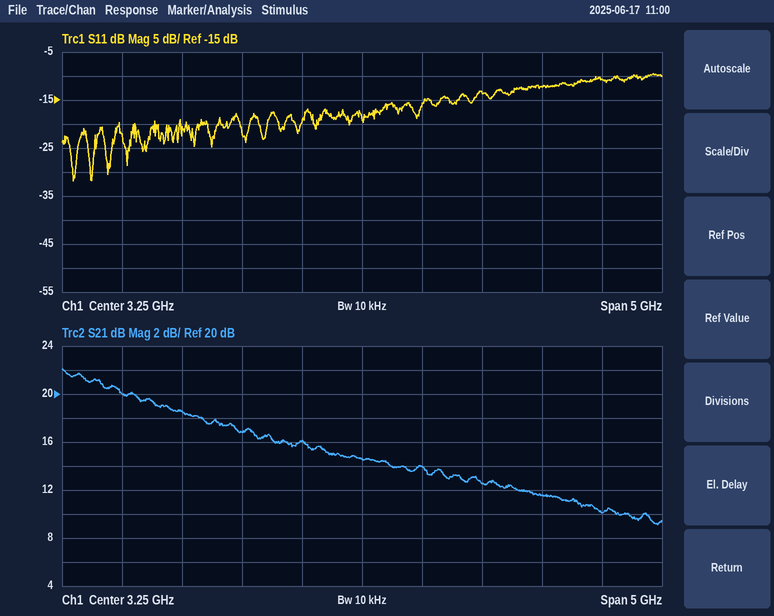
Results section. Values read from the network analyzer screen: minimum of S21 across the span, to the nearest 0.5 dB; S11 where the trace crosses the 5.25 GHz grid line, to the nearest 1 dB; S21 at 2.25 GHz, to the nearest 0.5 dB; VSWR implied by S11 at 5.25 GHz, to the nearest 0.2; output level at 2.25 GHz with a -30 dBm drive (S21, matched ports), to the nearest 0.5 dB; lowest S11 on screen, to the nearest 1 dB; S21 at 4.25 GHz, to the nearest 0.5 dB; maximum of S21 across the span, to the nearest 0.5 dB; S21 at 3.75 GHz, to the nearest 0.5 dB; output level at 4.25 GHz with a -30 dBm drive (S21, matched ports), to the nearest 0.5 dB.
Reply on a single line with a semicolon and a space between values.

9.0 dB; -11 dB; 17.0 dB; 1.8; -13.0 dBm; -32 dB; 12.5 dB; 22.0 dB; 14.0 dB; -17.5 dBm
